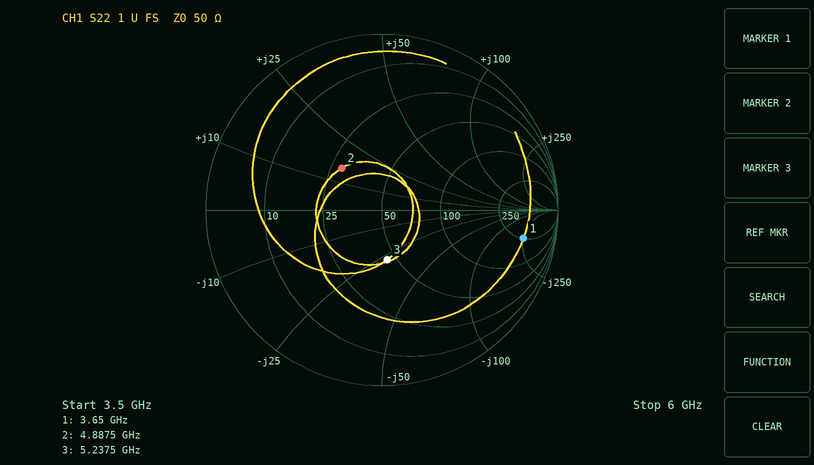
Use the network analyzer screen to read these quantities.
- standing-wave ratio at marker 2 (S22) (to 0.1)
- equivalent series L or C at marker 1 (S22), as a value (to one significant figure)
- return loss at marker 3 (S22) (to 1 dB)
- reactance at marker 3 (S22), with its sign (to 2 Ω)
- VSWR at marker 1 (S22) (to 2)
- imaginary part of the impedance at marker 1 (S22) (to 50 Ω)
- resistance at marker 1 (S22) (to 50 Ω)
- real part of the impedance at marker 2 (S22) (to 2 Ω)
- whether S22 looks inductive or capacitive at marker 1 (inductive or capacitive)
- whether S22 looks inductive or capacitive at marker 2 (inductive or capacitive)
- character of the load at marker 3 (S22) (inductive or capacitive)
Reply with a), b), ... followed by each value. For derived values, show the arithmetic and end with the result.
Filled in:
a) 2.0
b) C = 1/(2π × 3.65 GHz × 250 Ω) ≈ 174 fF, so 200 fF to one significant figure
c) 11 dB
d) -28 Ω
e) 10
f) -250 Ω
g) 250 Ω
h) 28 Ω
i) capacitive
j) inductive
k) capacitive
